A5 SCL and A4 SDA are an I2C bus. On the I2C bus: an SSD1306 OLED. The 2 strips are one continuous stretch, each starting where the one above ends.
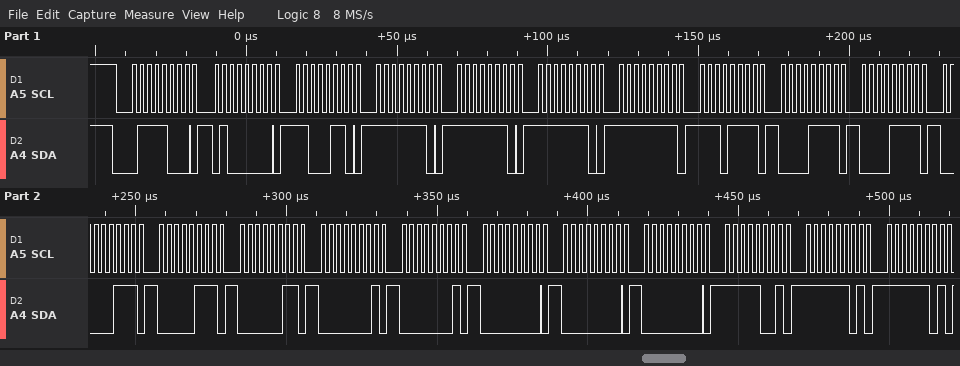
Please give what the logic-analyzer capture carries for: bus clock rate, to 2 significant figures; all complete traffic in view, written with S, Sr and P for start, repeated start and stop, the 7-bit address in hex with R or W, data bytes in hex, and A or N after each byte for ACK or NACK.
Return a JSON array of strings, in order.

["400 kHz", "S 3CW A 40 A C6 A FE A FE A FE A FF A EF A 0F A 0F A 07 A 07 A 03 A 01 A 01 A 00 A 00 A 00 A F9 A FD A FD A"]
